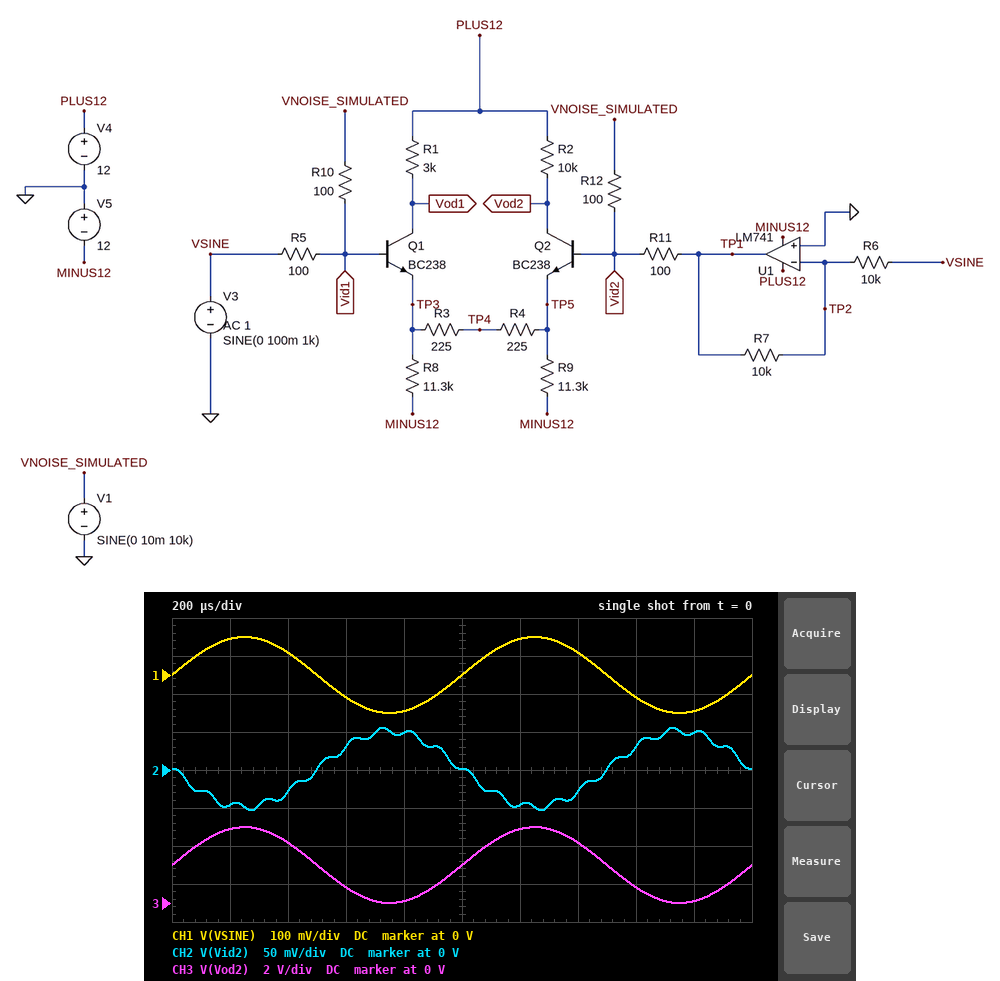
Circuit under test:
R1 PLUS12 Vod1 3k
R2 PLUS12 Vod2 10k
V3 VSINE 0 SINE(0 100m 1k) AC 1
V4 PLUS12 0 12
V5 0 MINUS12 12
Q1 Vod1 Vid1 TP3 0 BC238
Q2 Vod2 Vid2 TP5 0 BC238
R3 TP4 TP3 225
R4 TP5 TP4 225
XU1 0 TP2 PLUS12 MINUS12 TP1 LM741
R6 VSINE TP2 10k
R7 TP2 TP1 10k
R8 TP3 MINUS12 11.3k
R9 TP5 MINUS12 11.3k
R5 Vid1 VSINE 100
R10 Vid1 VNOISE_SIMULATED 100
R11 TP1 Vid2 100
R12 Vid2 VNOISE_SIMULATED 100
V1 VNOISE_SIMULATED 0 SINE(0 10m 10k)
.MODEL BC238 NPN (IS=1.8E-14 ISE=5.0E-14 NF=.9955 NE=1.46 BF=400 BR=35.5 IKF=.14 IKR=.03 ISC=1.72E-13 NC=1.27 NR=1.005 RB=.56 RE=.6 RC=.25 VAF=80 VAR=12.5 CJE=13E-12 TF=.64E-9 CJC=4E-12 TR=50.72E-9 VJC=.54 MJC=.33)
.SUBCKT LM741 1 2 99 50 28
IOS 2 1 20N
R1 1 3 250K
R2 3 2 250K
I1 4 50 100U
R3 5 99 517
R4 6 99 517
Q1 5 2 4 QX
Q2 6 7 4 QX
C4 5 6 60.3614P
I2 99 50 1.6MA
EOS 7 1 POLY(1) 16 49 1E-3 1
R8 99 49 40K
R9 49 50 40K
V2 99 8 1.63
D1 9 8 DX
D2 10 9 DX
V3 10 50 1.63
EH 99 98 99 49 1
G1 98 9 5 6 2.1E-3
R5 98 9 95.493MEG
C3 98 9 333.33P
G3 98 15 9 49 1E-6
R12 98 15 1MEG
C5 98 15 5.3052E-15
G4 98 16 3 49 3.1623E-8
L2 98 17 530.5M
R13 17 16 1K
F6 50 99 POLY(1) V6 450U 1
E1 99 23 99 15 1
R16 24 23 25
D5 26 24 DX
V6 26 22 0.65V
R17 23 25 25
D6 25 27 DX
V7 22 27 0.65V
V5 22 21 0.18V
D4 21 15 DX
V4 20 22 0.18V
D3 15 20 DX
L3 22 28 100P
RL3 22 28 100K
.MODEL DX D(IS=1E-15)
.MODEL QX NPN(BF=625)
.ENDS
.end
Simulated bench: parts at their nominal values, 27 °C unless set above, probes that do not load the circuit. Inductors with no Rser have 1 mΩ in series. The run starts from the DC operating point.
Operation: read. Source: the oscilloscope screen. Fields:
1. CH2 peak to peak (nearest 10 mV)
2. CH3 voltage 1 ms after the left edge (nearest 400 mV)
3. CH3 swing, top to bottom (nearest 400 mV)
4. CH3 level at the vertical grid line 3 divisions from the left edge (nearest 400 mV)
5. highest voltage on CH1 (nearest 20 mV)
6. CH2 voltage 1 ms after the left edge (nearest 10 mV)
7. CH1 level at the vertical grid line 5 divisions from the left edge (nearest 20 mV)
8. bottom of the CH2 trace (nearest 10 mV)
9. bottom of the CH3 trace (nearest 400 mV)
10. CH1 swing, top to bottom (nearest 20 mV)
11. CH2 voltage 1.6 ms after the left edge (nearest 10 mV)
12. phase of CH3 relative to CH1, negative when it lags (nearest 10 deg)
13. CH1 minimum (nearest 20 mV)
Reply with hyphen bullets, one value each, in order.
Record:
- 110 mV
- 2.0 V
- 4.0 V
- 800 mV
- 100 mV
- 0 V
- 0 V
- -50 mV
- 0 V
- 200 mV
- 30 mV
- 0 deg
- -100 mV
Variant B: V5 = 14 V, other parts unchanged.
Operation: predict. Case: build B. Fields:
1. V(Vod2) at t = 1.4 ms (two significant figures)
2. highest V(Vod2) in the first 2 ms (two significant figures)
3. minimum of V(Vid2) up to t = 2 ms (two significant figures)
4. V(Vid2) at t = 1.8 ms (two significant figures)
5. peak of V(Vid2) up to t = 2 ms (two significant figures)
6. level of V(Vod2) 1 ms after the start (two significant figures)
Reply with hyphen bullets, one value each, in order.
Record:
- 1.4 V
- 2.3 V
- -53 mV
- 45 mV
- 52 mV
- 240 mV
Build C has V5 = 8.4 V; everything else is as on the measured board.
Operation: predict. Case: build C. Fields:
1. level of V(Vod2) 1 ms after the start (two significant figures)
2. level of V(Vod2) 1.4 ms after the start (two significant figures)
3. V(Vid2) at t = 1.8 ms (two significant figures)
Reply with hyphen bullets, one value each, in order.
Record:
- 5.1 V
- 6.3 V
- 49 mV
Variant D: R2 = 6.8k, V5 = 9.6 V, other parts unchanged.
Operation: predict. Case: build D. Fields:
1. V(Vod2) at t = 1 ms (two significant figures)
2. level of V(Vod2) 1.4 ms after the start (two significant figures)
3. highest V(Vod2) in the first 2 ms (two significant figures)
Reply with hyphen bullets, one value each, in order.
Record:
- 6.6 V
- 7.4 V
- 7.9 V
